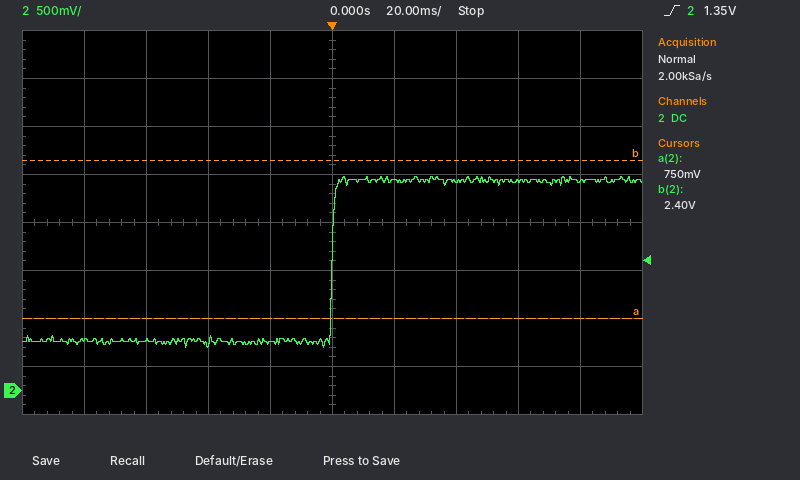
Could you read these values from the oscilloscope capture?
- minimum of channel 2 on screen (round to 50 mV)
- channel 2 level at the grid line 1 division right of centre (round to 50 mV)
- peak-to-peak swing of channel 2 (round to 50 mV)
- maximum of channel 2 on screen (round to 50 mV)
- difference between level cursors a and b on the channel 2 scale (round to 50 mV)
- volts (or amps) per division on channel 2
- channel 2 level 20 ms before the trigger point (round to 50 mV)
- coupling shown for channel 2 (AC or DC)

450 mV
2.20 V
1.80 V
2.25 V
1.65 V
500 mV
500 mV
DC
